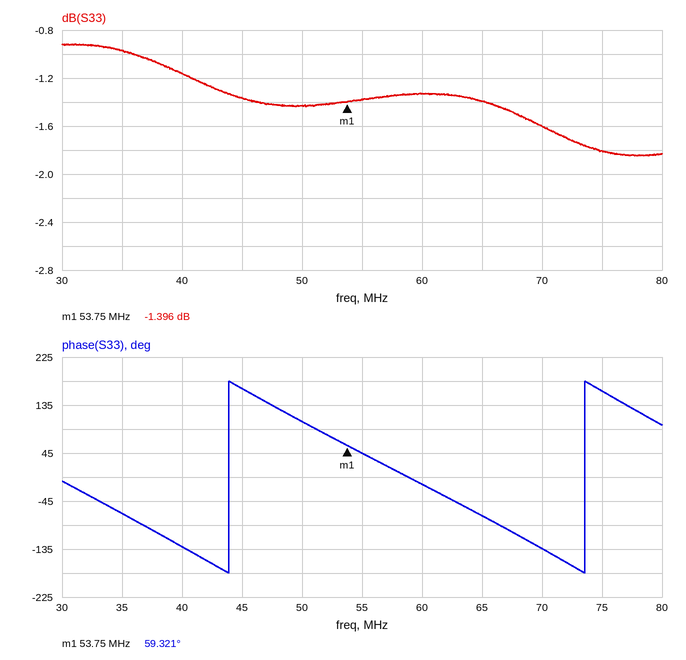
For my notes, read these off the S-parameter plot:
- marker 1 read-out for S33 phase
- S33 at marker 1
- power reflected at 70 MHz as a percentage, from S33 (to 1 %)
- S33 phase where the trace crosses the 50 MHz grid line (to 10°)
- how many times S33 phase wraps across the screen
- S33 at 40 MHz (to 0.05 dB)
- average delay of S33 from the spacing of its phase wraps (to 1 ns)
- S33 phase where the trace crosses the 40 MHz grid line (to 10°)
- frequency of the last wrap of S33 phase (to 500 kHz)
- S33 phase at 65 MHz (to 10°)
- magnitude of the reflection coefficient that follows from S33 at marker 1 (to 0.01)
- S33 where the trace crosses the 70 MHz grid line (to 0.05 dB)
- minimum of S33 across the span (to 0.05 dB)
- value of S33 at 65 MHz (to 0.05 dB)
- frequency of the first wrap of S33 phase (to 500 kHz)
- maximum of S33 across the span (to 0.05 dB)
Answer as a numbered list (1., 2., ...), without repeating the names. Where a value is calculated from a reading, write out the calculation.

1. 59.321°
2. -1.396 dB
3. 10^(-1.6/10) ≈ 69 %
4. 100°
5. 2
6. -1.15 dB
7. 1 cycle / (73.5 MHz − 44.0 MHz) ≈ 34 ns
8. -130°
9. 73.5 MHz
10. -70°
11. 10^(-1.396/20) ≈ 0.85
12. -1.60 dB
13. -1.85 dB
14. -1.40 dB
15. 44.0 MHz
16. -0.90 dB
